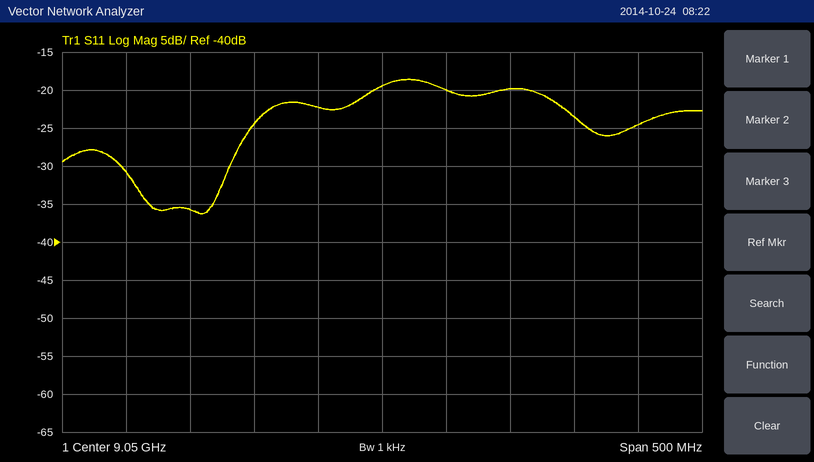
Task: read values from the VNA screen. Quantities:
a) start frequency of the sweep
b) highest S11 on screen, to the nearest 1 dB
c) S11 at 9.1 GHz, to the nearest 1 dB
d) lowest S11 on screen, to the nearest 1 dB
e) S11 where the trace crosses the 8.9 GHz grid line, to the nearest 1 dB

8.8 GHz
-19 dB
-20 dB
-36 dB
-36 dB
